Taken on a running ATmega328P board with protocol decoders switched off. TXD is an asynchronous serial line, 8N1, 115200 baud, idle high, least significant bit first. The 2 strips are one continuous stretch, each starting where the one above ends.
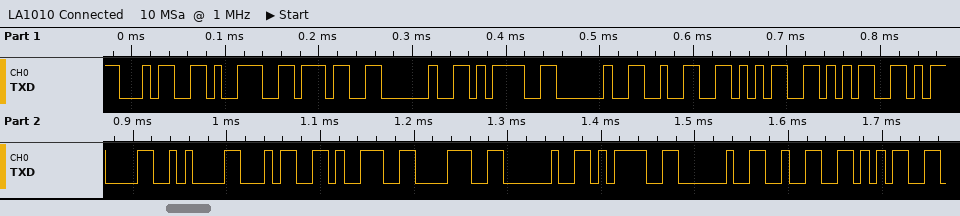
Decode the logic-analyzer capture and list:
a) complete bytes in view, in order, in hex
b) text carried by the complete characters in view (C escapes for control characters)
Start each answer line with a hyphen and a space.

- 34 39 37 20 3D 20 32 35 35 0D 0A 34 39 38 20 3D 20 32 35
- "497 = 255\r\n498 = 25"
